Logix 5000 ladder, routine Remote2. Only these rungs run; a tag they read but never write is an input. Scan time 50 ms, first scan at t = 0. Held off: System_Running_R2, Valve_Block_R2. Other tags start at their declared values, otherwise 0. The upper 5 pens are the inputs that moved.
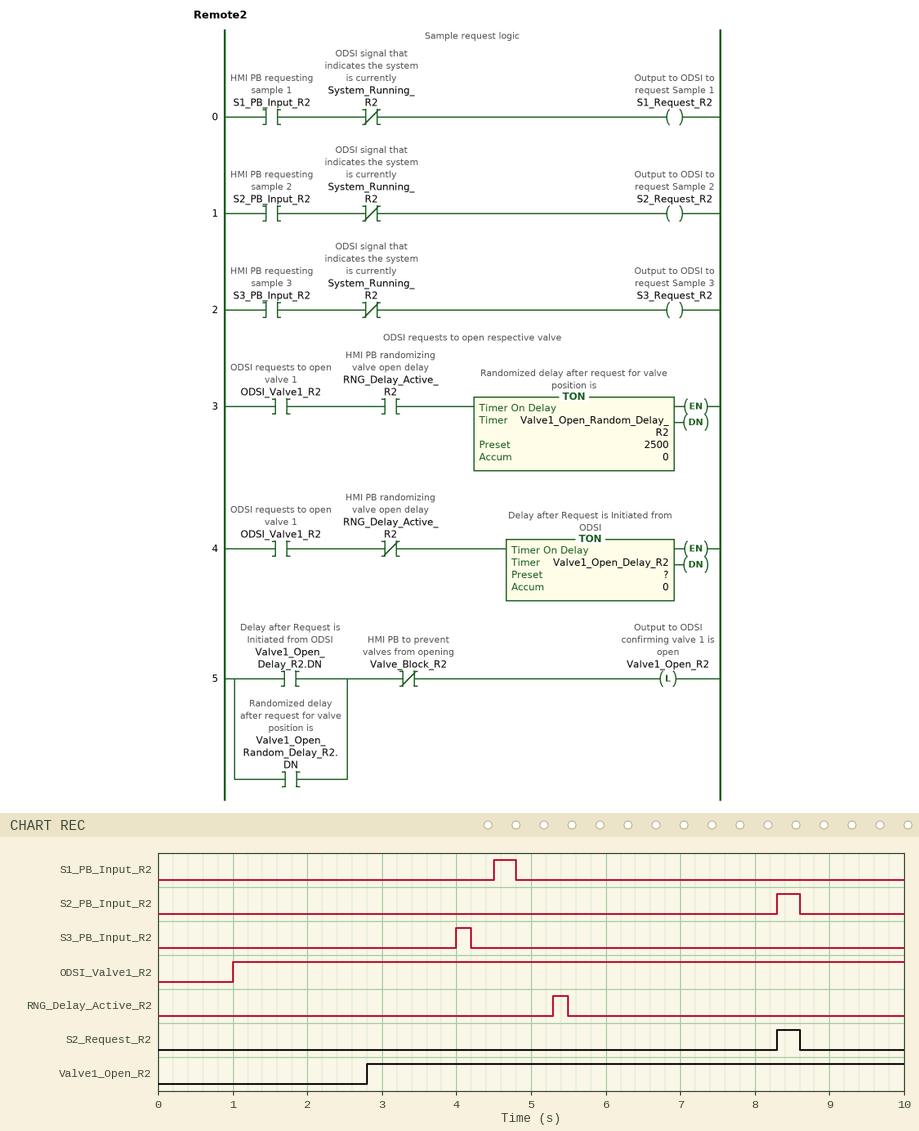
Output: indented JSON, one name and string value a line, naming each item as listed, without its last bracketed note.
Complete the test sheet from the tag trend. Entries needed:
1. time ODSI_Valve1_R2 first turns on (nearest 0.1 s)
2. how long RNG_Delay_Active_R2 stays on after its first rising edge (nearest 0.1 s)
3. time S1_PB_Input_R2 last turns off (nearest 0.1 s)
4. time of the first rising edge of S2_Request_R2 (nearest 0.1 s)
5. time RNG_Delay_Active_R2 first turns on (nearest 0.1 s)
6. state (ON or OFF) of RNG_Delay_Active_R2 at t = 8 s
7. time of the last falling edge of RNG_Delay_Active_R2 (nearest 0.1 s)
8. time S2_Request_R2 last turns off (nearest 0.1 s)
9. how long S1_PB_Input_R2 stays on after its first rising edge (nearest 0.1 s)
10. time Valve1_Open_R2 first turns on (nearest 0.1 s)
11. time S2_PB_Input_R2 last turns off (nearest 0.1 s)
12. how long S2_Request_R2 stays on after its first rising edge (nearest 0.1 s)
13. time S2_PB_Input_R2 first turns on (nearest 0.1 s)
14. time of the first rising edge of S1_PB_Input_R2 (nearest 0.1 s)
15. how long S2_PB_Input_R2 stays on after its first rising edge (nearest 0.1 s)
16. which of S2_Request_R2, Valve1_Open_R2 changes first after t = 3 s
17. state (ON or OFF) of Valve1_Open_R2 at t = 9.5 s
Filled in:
{
  "time ODSI_Valve1_R2 first turns on": "1.0 s",
  "how long RNG_Delay_Active_R2 stays on after its first rising edge": "0.2 s",
  "time S1_PB_Input_R2 last turns off": "4.8 s",
  "time of the first rising edge of S2_Request_R2": "8.3 s",
  "time RNG_Delay_Active_R2 first turns on": "5.3 s",
  "state (ON or OFF) of RNG_Delay_Active_R2 at t = 8 s": "OFF",
  "time of the last falling edge of RNG_Delay_Active_R2": "5.5 s",
  "time S2_Request_R2 last turns off": "8.6 s",
  "how long S1_PB_Input_R2 stays on after its first rising edge": "0.3 s",
  "time Valve1_Open_R2 first turns on": "2.8 s",
  "time S2_PB_Input_R2 last turns off": "8.6 s",
  "how long S2_Request_R2 stays on after its first rising edge": "0.3 s",
  "time S2_PB_Input_R2 first turns on": "8.3 s",
  "time of the first rising edge of S1_PB_Input_R2": "4.5 s",
  "how long S2_PB_Input_R2 stays on after its first rising edge": "0.3 s",
  "which of S2_Request_R2, Valve1_Open_R2 changes first after t = 3 s": "S2_Request_R2",
  "state (ON or OFF) of Valve1_Open_R2 at t = 9.5 s": "ON"
}
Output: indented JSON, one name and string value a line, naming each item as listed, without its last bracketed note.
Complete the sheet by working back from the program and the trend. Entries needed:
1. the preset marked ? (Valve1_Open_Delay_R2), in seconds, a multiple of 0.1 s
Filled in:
{
  "the preset marked ? (Valve1_Open_Delay_R2), in seconds, a multiple of 0.1 s": "1.8 s"
}
